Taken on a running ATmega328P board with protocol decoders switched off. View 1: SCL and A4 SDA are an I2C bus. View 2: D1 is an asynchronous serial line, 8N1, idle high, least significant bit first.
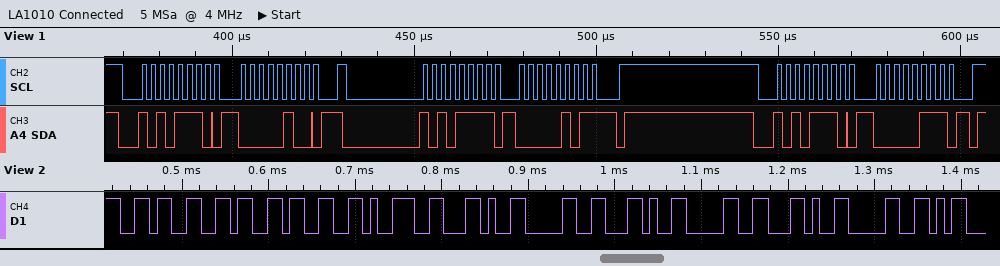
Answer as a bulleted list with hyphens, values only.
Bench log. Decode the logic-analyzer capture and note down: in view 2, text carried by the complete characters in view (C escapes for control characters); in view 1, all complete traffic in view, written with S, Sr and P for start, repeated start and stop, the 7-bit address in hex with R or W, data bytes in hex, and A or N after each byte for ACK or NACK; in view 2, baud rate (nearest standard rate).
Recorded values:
- "6639,0,0,0"
- S 57W A 04 A Sr 57R A 05 N P S 57W A 07 A P
- 115200 baud
